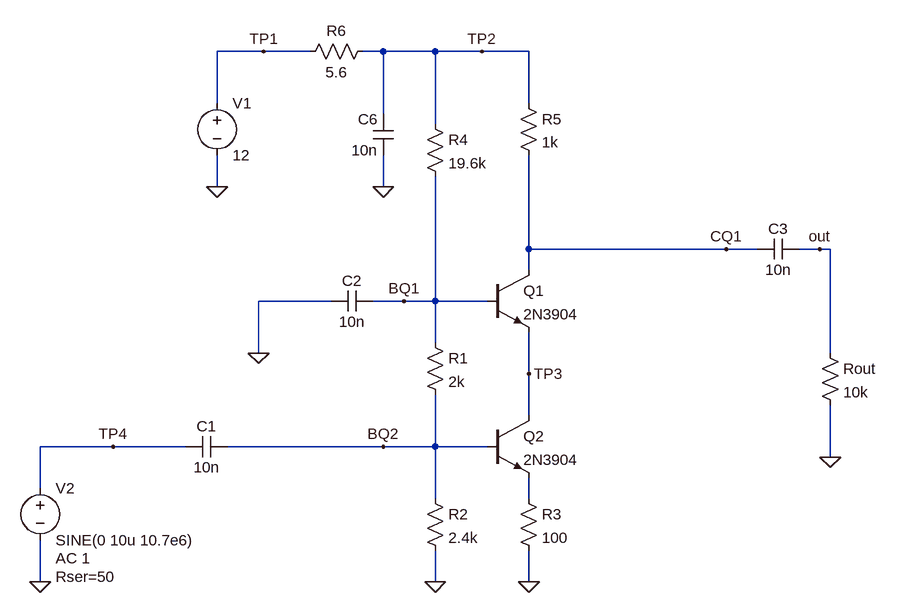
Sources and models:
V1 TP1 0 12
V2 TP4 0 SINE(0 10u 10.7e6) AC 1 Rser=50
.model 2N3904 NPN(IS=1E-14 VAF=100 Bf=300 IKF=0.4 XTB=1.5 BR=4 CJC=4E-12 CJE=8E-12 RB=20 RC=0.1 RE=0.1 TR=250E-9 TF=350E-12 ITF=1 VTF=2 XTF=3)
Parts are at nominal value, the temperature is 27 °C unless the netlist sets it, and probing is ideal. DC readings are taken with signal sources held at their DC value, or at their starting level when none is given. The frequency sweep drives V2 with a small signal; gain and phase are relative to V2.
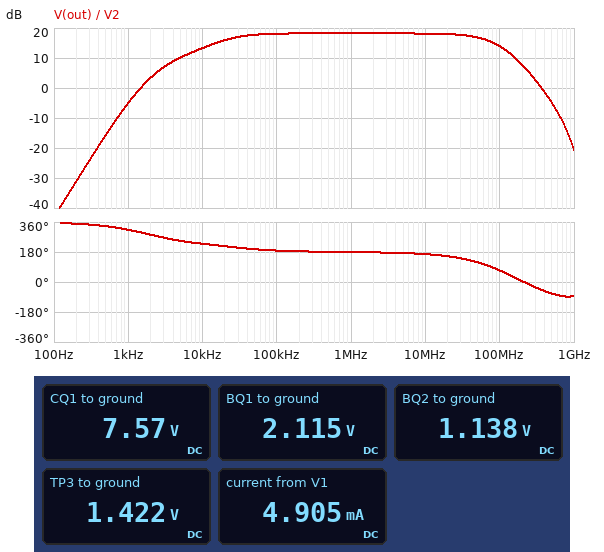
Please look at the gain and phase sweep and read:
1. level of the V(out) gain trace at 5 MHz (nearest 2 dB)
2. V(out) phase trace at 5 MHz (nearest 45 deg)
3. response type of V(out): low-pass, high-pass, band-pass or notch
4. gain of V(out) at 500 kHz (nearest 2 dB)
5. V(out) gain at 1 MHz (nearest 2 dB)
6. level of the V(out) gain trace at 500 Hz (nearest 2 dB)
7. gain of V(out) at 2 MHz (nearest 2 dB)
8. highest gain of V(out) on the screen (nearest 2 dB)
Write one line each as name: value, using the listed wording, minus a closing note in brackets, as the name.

level of the V(out) gain trace at 5 MHz: 18 dB
V(out) phase trace at 5 MHz: 180 deg
response type of V(out): low-pass, high-pass, band-pass or notch: band-pass
gain of V(out) at 500 kHz: 18 dB
V(out) gain at 1 MHz: 18 dB
level of the V(out) gain trace at 500 Hz: -16 dB
gain of V(out) at 2 MHz: 18 dB
highest gain of V(out) on the screen: 18 dB
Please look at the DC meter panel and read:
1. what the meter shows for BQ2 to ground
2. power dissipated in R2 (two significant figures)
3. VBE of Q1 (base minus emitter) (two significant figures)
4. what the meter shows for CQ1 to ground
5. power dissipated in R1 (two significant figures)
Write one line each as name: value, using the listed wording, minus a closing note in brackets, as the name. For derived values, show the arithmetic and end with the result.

what the meter shows for BQ2 to ground: 1.138 V
power dissipated in R2: (1.138 V)^2 / 2.4 kΩ = 540 µW
VBE of Q1 (base minus emitter): 2.115 V - 1.422 V = 690 mV
what the meter shows for CQ1 to ground: 7.57 V
power dissipated in R1: (2.115 V - 1.138 V)^2 / 2 kΩ = 480 µW
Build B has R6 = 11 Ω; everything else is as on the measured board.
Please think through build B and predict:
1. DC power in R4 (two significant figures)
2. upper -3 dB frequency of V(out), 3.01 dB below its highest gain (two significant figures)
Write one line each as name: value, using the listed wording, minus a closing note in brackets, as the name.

DC power in R4: 4.9 mW
upper -3 dB frequency of V(out), 3.01 dB below its highest gain: 79 MHz
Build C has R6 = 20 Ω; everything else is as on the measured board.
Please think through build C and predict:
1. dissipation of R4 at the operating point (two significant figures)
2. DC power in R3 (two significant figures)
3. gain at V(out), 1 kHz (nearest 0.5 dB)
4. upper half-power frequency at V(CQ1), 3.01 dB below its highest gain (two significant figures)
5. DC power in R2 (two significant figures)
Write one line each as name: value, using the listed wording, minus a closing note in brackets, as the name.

dissipation of R4 at the operating point: 4.9 mW
DC power in R3: 1.9 mW
gain at V(out), 1 kHz: -5.0 dB
upper half-power frequency at V(CQ1), 3.01 dB below its highest gain: 78 MHz
DC power in R2: 530 µW
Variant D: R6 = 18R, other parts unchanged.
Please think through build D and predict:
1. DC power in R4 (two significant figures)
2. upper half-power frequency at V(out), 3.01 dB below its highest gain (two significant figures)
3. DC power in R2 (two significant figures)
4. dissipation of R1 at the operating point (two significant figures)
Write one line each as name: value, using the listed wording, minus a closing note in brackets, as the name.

DC power in R4: 4.9 mW
upper half-power frequency at V(out), 3.01 dB below its highest gain: 78 MHz
DC power in R2: 530 µW
dissipation of R1 at the operating point: 470 µW
